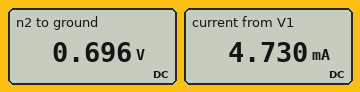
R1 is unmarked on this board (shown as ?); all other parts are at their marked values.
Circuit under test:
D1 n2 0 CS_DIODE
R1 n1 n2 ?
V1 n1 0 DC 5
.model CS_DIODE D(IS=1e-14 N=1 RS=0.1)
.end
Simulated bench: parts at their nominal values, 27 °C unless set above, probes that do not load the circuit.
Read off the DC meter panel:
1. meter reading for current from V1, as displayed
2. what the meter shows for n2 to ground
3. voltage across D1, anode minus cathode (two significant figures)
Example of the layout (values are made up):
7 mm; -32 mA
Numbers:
4.730 mA; 0.696 V; 700 mV
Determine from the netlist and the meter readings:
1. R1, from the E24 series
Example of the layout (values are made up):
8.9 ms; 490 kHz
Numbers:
910 Ω
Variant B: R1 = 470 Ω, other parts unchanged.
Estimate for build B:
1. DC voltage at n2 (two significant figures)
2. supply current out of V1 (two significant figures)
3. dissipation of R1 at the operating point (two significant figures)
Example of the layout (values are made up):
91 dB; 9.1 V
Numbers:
710 mV; 9.1 mA; 39 mW
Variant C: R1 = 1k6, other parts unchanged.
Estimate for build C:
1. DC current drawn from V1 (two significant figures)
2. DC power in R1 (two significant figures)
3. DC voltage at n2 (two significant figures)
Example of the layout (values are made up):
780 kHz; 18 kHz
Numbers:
2.7 mA; 12 mW; 680 mV
